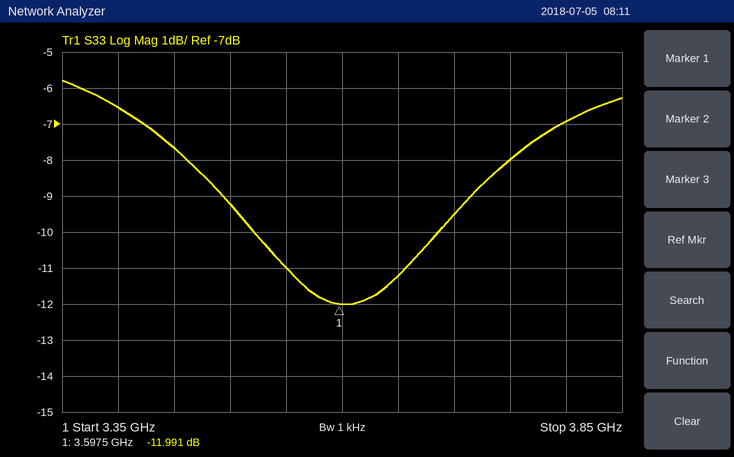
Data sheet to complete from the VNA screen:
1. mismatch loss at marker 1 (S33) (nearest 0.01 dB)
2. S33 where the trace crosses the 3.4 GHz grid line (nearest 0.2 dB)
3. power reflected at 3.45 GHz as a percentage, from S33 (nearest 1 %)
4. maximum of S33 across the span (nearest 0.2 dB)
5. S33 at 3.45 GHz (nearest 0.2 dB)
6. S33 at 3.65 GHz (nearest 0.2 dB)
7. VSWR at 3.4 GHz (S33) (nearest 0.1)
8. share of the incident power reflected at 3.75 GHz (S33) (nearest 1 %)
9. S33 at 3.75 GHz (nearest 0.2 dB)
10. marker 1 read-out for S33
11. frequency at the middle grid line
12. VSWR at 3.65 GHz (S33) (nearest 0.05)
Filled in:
0.28 dB
-6.6 dB
17 %
-5.8 dB
-7.6 dB
-11.2 dB
2.8
16 %
-8.0 dB
-11.991 dB
3.6 GHz
1.75
